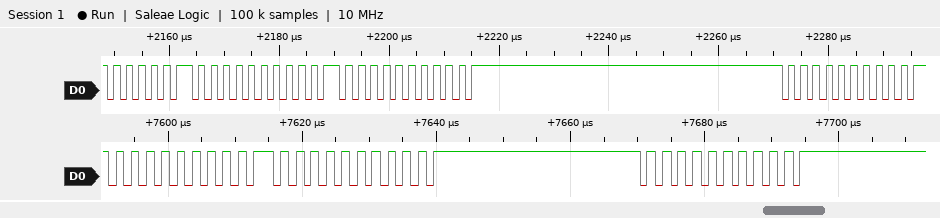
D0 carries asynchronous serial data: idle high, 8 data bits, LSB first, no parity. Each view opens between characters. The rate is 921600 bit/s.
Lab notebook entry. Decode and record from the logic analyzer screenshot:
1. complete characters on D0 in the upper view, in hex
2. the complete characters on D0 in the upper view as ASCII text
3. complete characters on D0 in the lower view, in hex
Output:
55, 57, 55, 75, 55, 55, 55, 55
"UWUuUUUU"
55, 55, 55, 55, FF, 55, 55, FF
